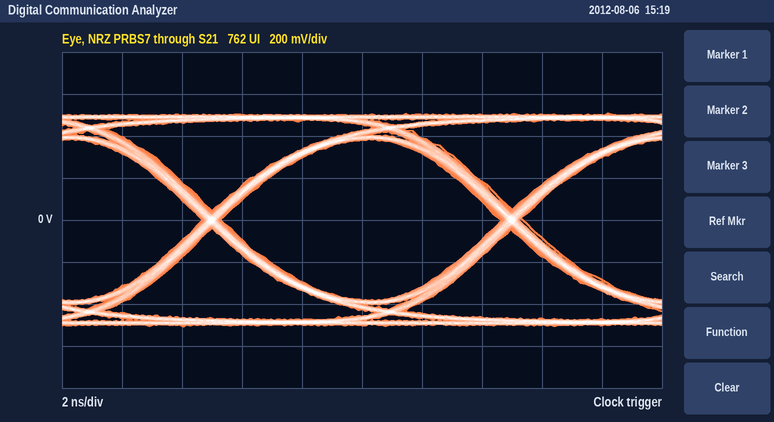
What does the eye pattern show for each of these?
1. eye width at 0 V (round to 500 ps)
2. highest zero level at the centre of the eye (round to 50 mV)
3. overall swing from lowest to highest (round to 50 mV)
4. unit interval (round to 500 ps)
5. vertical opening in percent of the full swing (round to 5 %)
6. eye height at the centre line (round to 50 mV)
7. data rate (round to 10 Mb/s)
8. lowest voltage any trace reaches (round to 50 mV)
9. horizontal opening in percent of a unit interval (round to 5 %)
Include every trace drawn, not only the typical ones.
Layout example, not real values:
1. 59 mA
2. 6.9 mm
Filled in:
1. 9.5 ns
2. -400 mV
3. 1.00 V
4. 10.0 ns
5. 75 %
6. 750 mV
7. 100 Mb/s
8. -500 mV
9. 95 %
